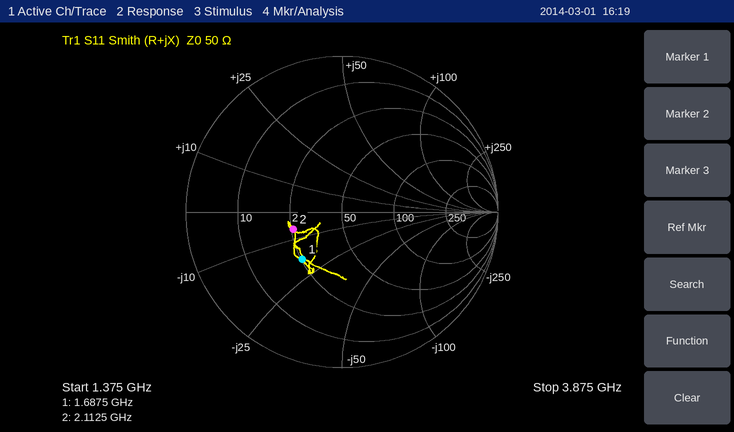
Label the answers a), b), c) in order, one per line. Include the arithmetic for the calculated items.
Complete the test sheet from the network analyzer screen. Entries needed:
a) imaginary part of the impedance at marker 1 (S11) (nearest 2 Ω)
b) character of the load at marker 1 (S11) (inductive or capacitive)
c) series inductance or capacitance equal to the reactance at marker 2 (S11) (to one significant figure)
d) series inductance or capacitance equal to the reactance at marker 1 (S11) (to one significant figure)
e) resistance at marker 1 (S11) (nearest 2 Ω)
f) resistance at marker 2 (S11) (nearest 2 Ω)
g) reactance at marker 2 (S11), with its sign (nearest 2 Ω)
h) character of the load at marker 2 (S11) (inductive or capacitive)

a) -18 Ω
b) capacitive
c) C = 1/(2π × 2.1125 GHz × 6 Ω) ≈ 12.6 pF, so 10 pF to one significant figure
d) C = 1/(2π × 1.6875 GHz × 18 Ω) ≈ 5 pF
e) 26 Ω
f) 26 Ω
g) -6 Ω
h) capacitive
